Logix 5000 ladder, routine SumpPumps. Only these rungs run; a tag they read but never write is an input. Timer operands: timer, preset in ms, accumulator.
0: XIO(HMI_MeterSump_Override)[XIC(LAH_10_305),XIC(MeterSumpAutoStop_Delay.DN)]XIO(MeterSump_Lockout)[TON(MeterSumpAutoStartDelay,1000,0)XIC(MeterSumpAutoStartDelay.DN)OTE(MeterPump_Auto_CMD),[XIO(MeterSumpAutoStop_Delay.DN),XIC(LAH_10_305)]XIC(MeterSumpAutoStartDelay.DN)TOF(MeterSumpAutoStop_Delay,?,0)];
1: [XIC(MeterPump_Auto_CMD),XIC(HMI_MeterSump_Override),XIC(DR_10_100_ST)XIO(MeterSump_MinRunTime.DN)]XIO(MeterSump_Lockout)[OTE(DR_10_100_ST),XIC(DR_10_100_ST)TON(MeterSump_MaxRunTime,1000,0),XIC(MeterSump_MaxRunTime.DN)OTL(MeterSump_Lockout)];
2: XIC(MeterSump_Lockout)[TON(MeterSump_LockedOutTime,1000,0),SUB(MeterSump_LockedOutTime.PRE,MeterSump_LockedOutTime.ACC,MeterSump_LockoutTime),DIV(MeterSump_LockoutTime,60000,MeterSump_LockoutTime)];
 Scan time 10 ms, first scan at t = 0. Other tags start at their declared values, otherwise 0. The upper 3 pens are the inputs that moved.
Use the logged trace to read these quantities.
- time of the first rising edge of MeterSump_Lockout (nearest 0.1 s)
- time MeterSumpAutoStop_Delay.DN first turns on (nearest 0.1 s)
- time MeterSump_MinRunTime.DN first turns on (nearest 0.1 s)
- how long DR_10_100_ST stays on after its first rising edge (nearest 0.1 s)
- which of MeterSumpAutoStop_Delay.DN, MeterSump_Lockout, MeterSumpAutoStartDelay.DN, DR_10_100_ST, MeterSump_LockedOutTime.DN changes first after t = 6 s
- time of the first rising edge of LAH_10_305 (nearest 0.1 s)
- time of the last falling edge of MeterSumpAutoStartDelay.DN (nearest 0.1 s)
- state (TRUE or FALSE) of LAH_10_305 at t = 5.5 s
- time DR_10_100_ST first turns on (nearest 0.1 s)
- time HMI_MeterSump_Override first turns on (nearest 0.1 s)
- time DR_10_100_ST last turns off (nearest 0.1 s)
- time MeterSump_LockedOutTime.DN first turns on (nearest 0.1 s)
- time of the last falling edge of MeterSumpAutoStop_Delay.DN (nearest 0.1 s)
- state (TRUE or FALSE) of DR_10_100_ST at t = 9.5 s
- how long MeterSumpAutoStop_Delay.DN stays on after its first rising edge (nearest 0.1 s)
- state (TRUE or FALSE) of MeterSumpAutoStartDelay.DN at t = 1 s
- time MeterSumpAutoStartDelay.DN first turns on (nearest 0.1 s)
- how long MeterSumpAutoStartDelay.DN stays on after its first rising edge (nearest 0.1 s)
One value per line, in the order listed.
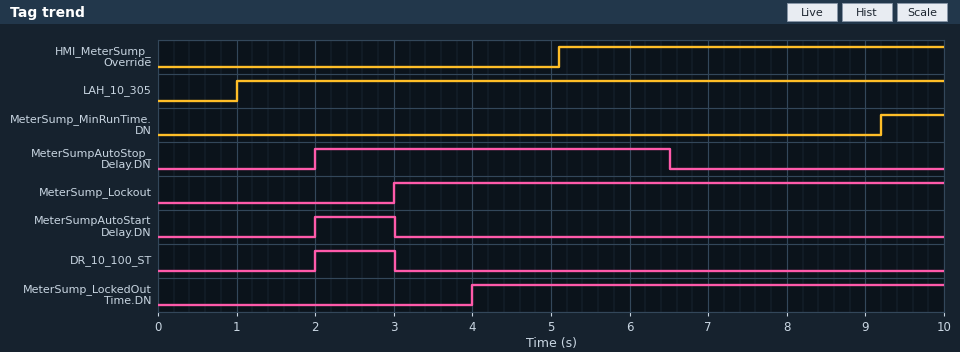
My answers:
3.0 s
2.0 s
9.2 s
1.0 s
MeterSumpAutoStop_Delay.DN
1.0 s
3.0 s
TRUE
2.0 s
5.1 s
3.0 s
4.0 s
6.5 s
FALSE
4.5 s
FALSE
2.0 s
1.0 s
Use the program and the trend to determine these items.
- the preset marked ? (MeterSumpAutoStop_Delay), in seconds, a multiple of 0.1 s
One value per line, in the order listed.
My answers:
3.5 s
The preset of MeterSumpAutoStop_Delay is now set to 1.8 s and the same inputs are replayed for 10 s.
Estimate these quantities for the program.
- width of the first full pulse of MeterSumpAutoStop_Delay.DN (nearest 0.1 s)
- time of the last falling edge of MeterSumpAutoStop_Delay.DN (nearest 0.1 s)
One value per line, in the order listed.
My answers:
2.8 s
4.8 s
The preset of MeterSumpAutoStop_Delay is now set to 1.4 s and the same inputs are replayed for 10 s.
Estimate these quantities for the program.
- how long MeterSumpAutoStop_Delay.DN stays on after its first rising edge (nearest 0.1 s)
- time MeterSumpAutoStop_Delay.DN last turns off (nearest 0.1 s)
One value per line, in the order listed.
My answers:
2.4 s
4.4 s
